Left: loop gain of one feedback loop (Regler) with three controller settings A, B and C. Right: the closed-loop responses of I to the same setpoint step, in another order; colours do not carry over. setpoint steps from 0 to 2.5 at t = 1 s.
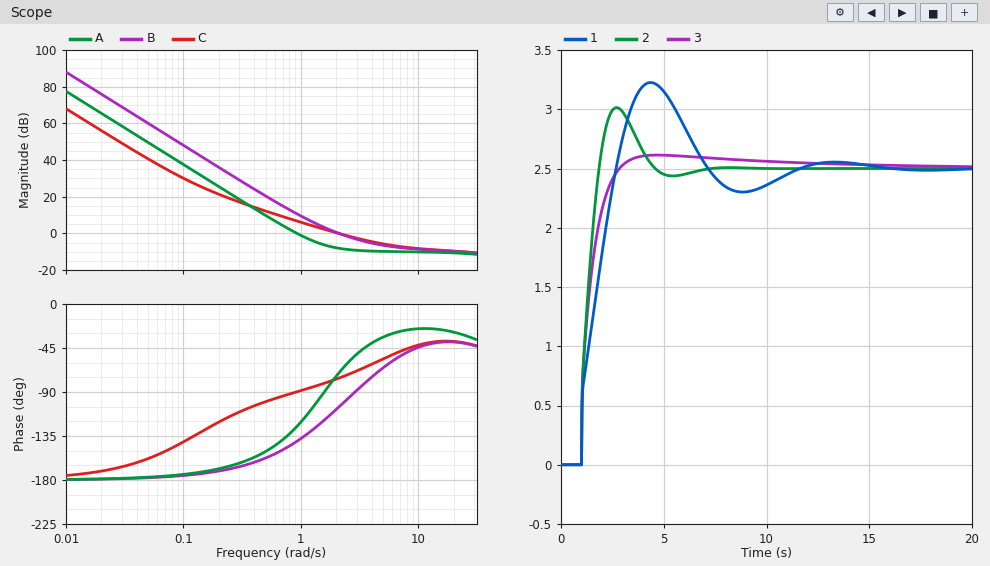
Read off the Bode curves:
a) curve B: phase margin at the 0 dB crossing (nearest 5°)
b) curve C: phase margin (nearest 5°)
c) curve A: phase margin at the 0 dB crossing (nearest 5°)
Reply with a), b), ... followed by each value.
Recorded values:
a) 75°
b) 105°
c) 55°
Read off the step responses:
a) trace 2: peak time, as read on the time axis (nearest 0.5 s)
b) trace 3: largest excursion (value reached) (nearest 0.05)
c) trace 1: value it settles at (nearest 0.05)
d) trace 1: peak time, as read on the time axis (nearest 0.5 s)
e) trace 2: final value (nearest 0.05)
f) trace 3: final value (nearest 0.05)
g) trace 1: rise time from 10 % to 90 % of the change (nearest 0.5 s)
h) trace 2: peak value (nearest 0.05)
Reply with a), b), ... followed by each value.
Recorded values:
a) 2.5 s
b) 2.60
c) 2.50
d) 4.5 s
e) 2.50
f) 2.50
g) 1.5 s
h) 3.00
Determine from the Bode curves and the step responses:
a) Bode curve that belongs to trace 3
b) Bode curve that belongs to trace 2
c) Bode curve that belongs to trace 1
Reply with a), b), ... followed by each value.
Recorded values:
a) C
b) B
c) A
